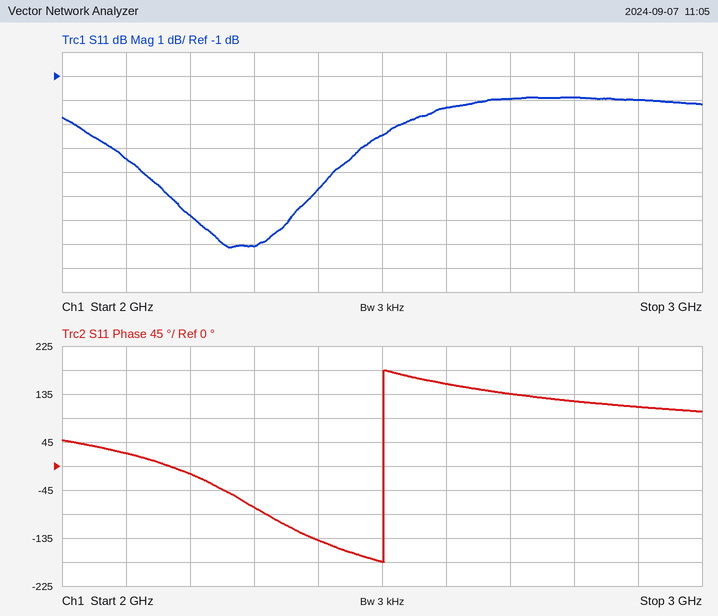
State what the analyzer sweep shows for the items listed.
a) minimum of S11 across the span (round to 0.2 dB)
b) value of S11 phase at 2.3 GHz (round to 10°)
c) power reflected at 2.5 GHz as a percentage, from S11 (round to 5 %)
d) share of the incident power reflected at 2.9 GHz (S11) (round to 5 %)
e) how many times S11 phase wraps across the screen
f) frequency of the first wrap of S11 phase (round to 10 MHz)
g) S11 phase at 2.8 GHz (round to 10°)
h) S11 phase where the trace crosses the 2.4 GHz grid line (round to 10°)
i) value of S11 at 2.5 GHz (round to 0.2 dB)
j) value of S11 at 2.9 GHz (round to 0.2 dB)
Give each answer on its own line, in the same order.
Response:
-8.2 dB
-80°
45 %
65 %
1
2.50 GHz
120°
-140°
-3.4 dB
-2.0 dB
